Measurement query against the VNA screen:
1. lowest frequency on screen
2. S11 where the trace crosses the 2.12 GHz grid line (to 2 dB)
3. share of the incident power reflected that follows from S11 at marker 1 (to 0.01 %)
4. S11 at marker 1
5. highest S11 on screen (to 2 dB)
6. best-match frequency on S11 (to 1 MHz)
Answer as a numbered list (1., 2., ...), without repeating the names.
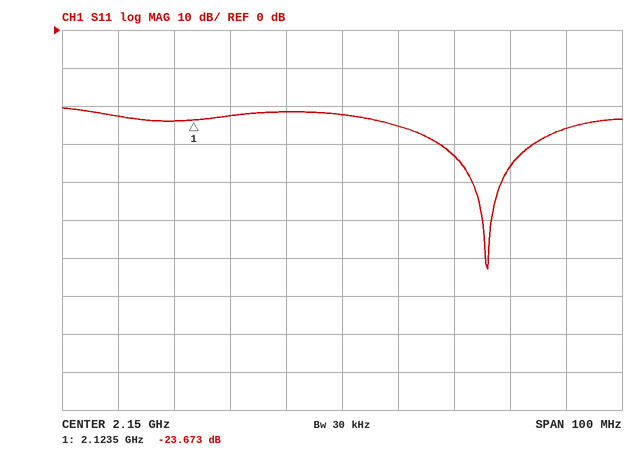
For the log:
1. 2.1 GHz
2. -24 dB
3. 0.43 %
4. -23.673 dB
5. -20 dB
6. 2.176 GHz
